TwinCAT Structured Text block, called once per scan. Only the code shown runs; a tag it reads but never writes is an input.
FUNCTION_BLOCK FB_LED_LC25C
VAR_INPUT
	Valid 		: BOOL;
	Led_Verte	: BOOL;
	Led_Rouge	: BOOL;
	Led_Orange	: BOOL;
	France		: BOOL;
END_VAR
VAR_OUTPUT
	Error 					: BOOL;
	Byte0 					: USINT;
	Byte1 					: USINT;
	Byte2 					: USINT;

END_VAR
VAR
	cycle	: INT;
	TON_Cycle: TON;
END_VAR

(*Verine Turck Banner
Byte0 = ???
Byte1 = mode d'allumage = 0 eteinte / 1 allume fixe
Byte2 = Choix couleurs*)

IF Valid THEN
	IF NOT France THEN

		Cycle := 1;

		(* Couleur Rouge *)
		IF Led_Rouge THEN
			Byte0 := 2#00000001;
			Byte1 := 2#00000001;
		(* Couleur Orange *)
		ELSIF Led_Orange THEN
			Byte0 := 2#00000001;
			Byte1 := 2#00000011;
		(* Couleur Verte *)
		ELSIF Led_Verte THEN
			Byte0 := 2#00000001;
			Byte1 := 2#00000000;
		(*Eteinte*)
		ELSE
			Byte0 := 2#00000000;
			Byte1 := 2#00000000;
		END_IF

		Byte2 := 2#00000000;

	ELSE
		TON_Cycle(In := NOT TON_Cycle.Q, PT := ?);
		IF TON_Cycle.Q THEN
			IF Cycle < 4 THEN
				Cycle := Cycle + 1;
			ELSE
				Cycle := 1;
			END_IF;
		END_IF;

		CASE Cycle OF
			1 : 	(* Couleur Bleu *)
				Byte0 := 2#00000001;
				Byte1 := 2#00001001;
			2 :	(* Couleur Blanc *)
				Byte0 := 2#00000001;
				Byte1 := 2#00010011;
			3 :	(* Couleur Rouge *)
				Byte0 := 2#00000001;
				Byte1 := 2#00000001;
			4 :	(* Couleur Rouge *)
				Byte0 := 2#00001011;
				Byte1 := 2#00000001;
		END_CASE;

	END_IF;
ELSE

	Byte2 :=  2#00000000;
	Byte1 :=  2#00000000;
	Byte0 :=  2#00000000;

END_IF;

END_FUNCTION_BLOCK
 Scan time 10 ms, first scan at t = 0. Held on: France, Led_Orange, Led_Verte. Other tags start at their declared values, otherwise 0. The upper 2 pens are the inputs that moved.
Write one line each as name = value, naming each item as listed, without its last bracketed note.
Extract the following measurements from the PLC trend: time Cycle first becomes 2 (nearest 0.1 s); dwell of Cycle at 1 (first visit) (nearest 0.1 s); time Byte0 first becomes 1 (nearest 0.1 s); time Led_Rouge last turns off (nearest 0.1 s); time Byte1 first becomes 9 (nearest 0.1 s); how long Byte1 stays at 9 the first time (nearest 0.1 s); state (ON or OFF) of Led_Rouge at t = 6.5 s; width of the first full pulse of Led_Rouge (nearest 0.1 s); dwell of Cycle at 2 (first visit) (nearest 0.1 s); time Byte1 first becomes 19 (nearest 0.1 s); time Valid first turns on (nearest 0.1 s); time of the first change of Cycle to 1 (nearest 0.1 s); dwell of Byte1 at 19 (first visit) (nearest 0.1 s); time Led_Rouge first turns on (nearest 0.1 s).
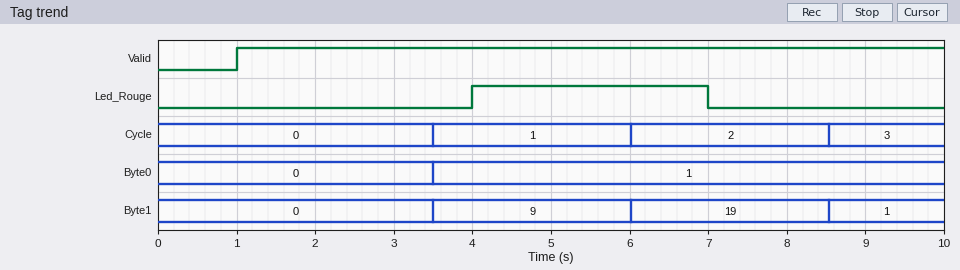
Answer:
time Cycle first becomes 2 = 6.0 s
dwell of Cycle at 1 (first visit) = 2.5 s
time Byte0 first becomes 1 = 3.5 s
time Led_Rouge last turns off = 7.0 s
time Byte1 first becomes 9 = 3.5 s
how long Byte1 stays at 9 the first time = 2.5 s
state (ON or OFF) of Led_Rouge at t = 6.5 s = ON
width of the first full pulse of Led_Rouge = 3.0 s
dwell of Cycle at 2 (first visit) = 2.5 s
time Byte1 first becomes 19 = 6.0 s
time Valid first turns on = 1.0 s
time of the first change of Cycle to 1 = 3.5 s
dwell of Byte1 at 19 (first visit) = 2.5 s
time Led_Rouge first turns on = 4.0 s
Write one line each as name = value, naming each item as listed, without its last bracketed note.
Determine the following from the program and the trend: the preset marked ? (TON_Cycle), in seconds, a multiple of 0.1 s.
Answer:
the preset marked ? (TON_Cycle), in seconds, a multiple of 0.1 s = 2.5 s
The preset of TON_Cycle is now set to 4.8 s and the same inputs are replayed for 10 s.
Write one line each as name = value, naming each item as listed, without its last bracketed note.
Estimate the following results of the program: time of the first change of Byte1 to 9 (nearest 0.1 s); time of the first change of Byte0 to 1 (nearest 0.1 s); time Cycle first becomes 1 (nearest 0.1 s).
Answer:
time of the first change of Byte1 to 9 = 5.8 s
time of the first change of Byte0 to 1 = 5.8 s
time Cycle first becomes 1 = 5.8 s
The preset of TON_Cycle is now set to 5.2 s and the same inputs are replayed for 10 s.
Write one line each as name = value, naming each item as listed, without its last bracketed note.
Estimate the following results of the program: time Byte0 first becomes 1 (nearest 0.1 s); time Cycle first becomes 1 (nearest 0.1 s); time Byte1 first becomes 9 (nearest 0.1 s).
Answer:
time Byte0 first becomes 1 = 6.2 s
time Cycle first becomes 1 = 6.2 s
time Byte1 first becomes 9 = 6.2 s
